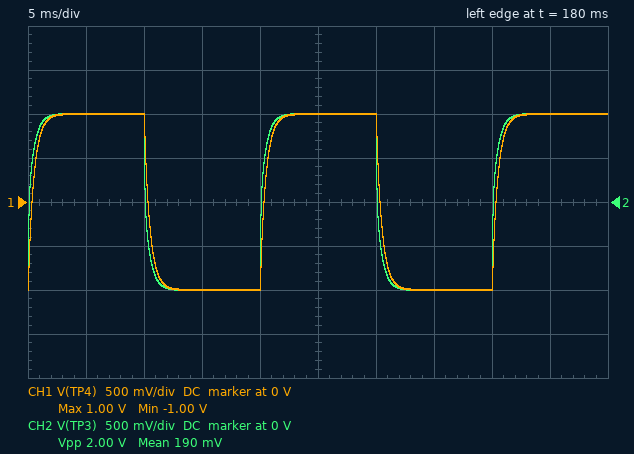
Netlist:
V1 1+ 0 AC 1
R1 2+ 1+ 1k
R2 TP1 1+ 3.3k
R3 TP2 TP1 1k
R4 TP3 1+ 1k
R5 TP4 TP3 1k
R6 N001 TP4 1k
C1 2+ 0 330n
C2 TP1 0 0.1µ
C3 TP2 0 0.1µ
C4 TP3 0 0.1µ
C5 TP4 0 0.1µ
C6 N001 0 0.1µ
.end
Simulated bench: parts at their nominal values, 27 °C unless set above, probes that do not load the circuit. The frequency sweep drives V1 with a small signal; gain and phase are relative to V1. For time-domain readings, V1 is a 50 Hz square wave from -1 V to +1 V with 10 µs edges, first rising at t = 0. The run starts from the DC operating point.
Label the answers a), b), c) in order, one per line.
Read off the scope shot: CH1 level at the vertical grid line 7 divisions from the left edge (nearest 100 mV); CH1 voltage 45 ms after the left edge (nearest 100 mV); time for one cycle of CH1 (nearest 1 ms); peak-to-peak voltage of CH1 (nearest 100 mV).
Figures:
a) -1.0 V
b) 1.0 V
c) 20 ms
d) 2.0 V
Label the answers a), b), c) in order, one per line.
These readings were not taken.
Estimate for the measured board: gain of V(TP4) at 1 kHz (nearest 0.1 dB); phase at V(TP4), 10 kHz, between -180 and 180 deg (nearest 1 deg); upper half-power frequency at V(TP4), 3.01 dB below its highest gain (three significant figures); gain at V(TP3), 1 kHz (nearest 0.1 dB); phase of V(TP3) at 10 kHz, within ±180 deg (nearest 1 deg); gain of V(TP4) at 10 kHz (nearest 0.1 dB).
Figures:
a) -9.8 dB
b) -146 deg
c) 321 Hz
d) -5.3 dB
e) -73 deg
f) -33.1 dB
